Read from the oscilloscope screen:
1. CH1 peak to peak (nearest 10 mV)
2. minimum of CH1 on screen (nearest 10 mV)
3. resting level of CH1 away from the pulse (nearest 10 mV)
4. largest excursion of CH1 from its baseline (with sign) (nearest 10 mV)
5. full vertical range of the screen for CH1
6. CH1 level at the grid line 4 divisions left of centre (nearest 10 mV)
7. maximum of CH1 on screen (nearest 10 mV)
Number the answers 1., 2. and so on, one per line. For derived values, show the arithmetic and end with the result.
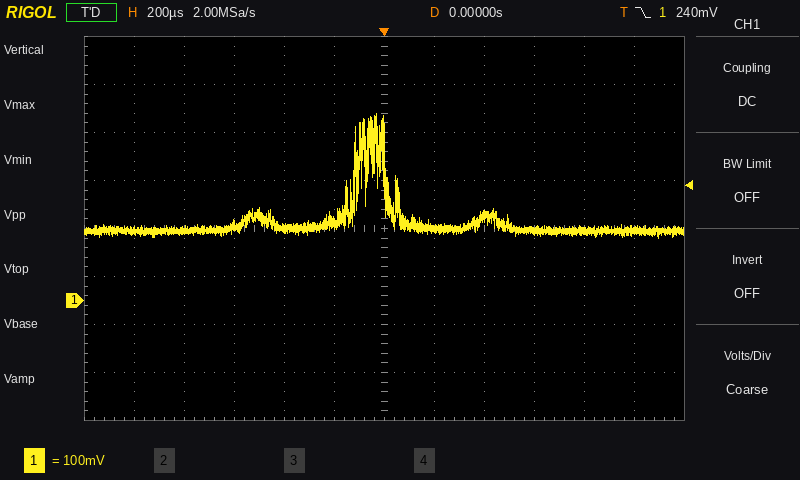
1. 390 mV − (130 mV) = 260 mV
2. 130 mV
3. 150 mV
4. 390 mV − (150 mV) = +240 mV
5. 800 mV
6. 150 mV
7. 390 mV
